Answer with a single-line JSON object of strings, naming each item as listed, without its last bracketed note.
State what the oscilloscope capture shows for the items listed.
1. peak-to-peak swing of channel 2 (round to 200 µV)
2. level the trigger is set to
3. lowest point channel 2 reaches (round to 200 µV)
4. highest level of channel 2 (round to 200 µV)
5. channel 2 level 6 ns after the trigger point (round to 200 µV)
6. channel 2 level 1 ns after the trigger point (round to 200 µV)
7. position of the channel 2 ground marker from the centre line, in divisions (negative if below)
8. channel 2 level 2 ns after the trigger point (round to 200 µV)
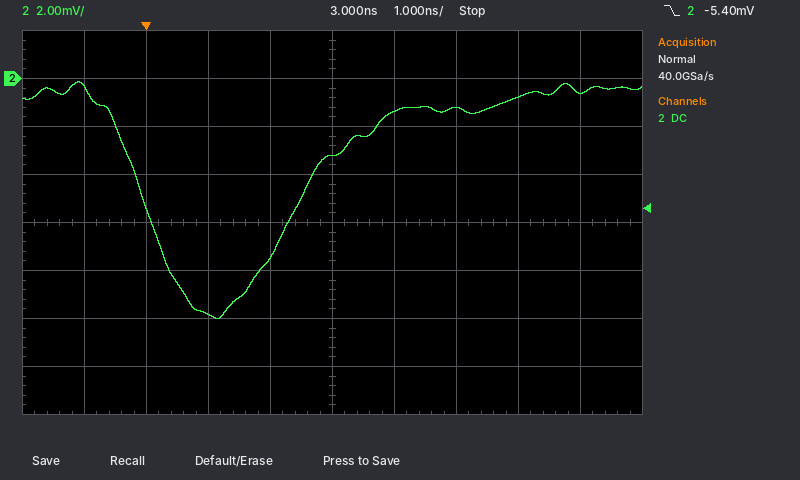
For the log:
{"peak-to-peak swing of channel 2": "9.8 mV", "level the trigger is set to": "-5.40 mV", "lowest point channel 2 reaches": "-10.0 mV", "highest level of channel 2": "-200 µV", "channel 2 level 6 ns after the trigger point": "-800 µV", "channel 2 level 1 ns after the trigger point": "-9.8 mV", "position of the channel 2 ground marker from the centre line, in divisions": "+3.0 div", "channel 2 level 2 ns after the trigger point": "-7.4 mV"}
